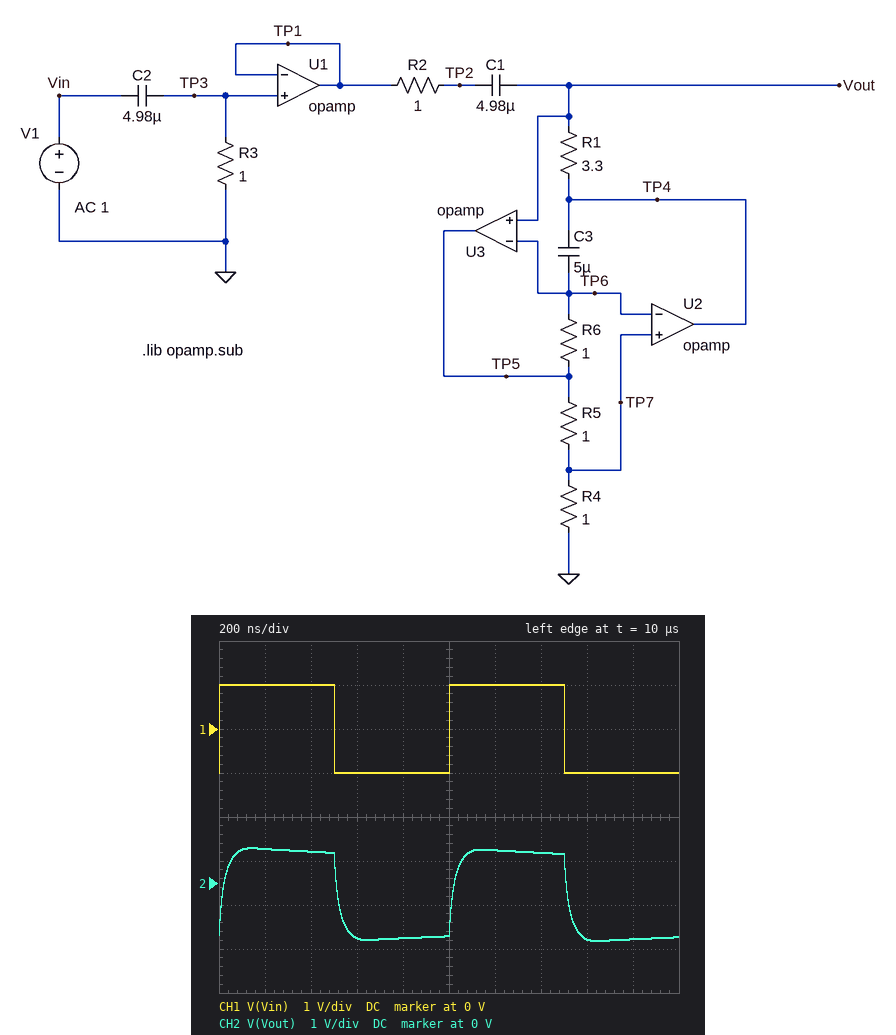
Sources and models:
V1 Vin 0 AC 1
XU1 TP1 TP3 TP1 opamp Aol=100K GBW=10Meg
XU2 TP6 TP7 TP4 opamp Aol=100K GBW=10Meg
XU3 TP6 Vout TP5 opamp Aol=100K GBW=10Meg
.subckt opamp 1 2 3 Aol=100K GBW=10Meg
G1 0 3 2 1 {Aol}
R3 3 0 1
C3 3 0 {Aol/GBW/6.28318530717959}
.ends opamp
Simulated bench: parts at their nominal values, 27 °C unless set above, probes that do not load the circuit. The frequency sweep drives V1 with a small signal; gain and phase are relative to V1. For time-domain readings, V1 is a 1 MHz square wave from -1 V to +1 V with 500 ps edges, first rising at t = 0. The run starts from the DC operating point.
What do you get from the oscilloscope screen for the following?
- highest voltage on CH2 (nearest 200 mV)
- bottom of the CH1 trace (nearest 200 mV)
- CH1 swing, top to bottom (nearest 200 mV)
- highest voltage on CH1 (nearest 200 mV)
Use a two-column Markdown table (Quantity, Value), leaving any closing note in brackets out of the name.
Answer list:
| Quantity | Value |
|---|---|
| highest voltage on CH2 | 800 mV |
| bottom of the CH1 trace | -1.0 V |
| CH1 swing, top to bottom | 2.0 V |
| highest voltage on CH1 | 1.0 V |
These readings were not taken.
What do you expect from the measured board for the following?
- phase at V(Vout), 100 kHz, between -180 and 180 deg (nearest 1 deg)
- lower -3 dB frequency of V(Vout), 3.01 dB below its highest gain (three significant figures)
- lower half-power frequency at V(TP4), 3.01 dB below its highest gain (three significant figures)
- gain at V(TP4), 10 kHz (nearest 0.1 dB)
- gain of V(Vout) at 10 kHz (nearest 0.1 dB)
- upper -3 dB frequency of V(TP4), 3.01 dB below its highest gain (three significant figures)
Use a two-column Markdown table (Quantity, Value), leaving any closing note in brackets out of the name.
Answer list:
| Quantity | Value |
|---|---|
| phase at V(Vout), 100 kHz, between -180 and 180 deg | 22 deg |
| lower -3 dB frequency of V(Vout), 3.01 dB below its highest gain | 16.0 kHz |
| lower half-power frequency at V(TP4), 3.01 dB below its highest gain | 14.9 kHz |
| gain at V(TP4), 10 kHz | -7.2 dB |
| gain of V(Vout) at 10 kHz | -17.6 dB |
| upper -3 dB frequency of V(TP4), 3.01 dB below its highest gain | 30.7 kHz |
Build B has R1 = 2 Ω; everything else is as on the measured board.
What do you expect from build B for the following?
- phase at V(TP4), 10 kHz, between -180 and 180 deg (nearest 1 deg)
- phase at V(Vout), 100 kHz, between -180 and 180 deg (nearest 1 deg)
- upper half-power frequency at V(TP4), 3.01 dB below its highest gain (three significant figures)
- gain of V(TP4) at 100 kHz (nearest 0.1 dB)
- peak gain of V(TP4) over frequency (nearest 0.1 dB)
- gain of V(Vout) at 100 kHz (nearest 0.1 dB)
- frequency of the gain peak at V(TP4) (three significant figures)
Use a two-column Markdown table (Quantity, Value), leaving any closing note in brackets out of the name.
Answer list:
| Quantity | Value |
|---|---|
| phase at V(TP4), 10 kHz, between -180 and 180 deg | -56 deg |
| phase at V(Vout), 100 kHz, between -180 and 180 deg | 26 deg |
| upper half-power frequency at V(TP4), 3.01 dB below its highest gain | 72.5 kHz |
| gain of V(TP4) at 100 kHz | 0.3 dB |
| peak gain of V(TP4) over frequency | 3.6 dB |
| gain of V(Vout) at 100 kHz | -0.1 dB |
| frequency of the gain peak at V(TP4) | 25.9 kHz |
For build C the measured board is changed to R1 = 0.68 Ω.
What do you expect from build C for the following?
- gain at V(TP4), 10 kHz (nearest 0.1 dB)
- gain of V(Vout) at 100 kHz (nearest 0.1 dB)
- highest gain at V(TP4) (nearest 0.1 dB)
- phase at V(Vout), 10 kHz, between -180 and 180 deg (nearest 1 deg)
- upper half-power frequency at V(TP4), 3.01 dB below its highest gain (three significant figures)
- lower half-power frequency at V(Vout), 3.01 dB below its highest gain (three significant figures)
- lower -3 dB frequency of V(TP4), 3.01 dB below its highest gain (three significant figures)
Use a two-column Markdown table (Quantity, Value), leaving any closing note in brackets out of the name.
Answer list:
| Quantity | Value |
|---|---|
| gain at V(TP4), 10 kHz | -23.4 dB |
| gain of V(Vout) at 100 kHz | -0.1 dB |
| highest gain at V(TP4) | 0.3 dB |
| phase at V(Vout), 10 kHz, between -180 and 180 deg | -126 deg |
| upper half-power frequency at V(TP4), 3.01 dB below its highest gain | 2.20 MHz |
| lower half-power frequency at V(Vout), 3.01 dB below its highest gain | 41.4 kHz |
| lower -3 dB frequency of V(TP4), 3.01 dB below its highest gain | 34.7 kHz |
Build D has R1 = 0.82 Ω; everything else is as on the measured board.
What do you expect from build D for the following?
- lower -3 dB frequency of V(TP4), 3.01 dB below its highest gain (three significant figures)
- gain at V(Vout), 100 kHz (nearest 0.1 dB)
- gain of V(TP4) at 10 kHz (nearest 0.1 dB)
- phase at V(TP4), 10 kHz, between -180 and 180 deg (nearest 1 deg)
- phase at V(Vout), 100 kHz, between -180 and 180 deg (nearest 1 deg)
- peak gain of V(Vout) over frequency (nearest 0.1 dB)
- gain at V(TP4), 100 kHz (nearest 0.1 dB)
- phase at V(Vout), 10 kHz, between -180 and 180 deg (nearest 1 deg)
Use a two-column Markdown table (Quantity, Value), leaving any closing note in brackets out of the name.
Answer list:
| Quantity | Value |
|---|---|
| lower -3 dB frequency of V(TP4), 3.01 dB below its highest gain | 30.6 kHz |
| gain at V(Vout), 100 kHz | 0 dB |
| gain of V(TP4) at 10 kHz | -21.6 dB |
| phase at V(TP4), 10 kHz, between -180 and 180 deg | -54 deg |
| phase at V(Vout), 100 kHz, between -180 and 180 deg | 39 deg |
| peak gain of V(Vout) over frequency | 0 dB |
| gain at V(TP4), 100 kHz | 0.3 dB |
| phase at V(Vout), 10 kHz, between -180 and 180 deg | -126 deg |
